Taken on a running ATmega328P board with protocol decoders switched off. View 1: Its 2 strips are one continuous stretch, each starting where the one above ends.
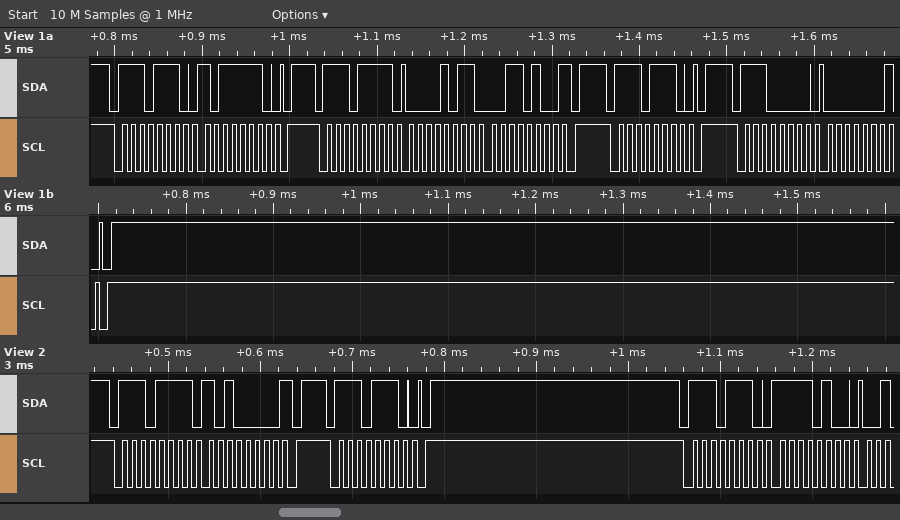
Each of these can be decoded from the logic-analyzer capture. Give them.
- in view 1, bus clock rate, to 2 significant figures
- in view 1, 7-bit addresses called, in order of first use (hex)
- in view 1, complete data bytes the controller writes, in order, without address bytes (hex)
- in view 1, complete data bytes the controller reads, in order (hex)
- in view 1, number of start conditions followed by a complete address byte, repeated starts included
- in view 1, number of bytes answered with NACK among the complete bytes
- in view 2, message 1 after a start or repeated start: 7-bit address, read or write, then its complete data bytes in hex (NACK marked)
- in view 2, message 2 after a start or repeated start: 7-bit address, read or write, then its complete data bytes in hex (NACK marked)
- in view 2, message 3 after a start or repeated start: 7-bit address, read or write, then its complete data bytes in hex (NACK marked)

100 kHz
0x77 0x70
BE 01
0B 34
4
1
0x77 read: A0 NACK
0x77 write
0x77 write: F4
